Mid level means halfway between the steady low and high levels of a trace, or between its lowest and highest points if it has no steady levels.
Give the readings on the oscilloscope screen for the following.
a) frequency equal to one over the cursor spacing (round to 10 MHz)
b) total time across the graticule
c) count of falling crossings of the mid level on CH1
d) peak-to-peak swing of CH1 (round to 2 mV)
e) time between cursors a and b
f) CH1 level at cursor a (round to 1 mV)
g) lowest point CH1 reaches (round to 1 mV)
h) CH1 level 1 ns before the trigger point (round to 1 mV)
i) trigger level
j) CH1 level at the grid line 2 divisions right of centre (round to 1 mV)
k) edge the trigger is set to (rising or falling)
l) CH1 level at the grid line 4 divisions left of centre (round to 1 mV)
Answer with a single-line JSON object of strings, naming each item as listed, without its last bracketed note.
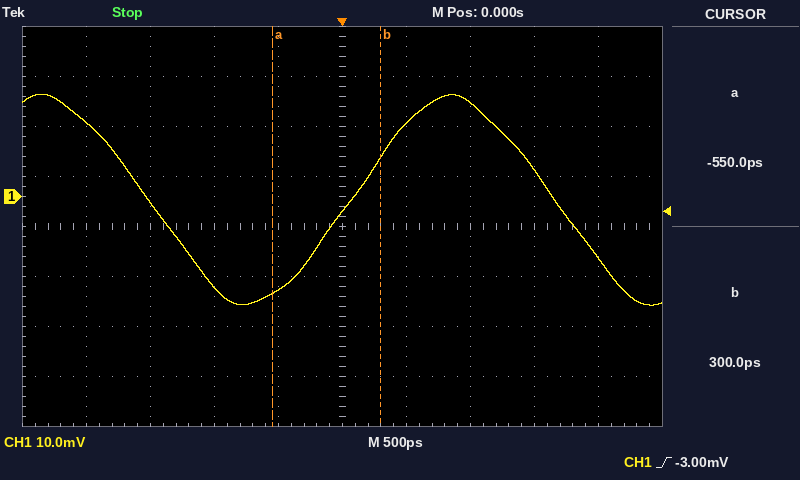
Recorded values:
{"frequency equal to one over the cursor spacing": "1.18 GHz", "total time across the graticule": "5 ns", "count of falling crossings of the mid level on CH1": "2", "peak-to-peak swing of CH1": "42 mV", "time between cursors a and b": "850 ps", "CH1 level at cursor a": "-19 mV", "lowest point CH1 reaches": "-22 mV", "CH1 level 1 ns before the trigger point": "-18 mV", "trigger level": "-3.00 mV", "CH1 level at the grid line 2 divisions right of centre": "19 mV", "edge the trigger is set to": "rising", "CH1 level at the grid line 4 divisions left of centre": "15 mV"}
